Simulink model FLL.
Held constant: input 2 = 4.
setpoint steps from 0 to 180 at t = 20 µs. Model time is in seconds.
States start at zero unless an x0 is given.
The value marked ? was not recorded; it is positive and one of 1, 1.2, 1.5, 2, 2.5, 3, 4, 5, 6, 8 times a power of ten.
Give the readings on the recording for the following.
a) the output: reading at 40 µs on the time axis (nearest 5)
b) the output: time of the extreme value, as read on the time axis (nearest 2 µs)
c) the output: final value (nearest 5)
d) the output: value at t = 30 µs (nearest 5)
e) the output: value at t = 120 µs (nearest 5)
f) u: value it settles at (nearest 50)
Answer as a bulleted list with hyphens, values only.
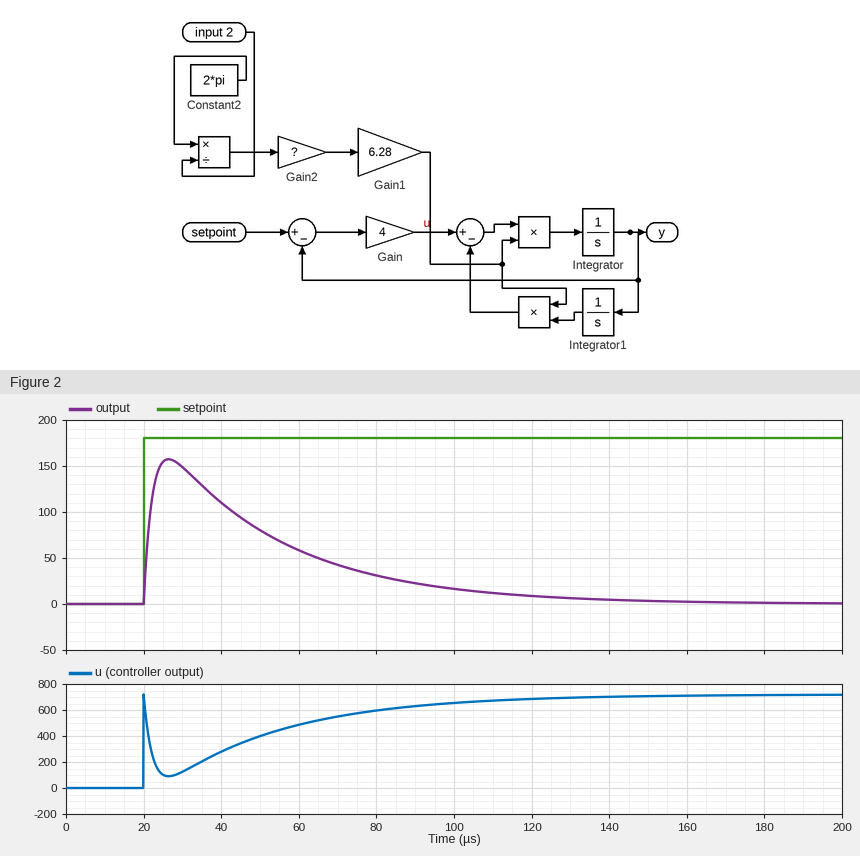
- 110
- 26 µs
- 0
- 150
- 10
- 700
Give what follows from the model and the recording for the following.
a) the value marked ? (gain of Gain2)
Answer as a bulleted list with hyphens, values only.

- 12000
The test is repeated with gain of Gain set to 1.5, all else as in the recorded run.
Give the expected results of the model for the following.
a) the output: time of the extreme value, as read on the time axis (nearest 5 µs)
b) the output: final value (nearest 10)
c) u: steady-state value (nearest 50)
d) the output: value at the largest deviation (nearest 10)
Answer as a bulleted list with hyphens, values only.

- 30 µs
- 0
- 250
- 120
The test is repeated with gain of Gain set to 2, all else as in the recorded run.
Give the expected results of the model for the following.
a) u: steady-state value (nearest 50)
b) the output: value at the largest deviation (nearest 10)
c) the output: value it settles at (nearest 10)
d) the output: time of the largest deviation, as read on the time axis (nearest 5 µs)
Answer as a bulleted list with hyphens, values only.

- 350
- 130
- 0
- 30 µs
